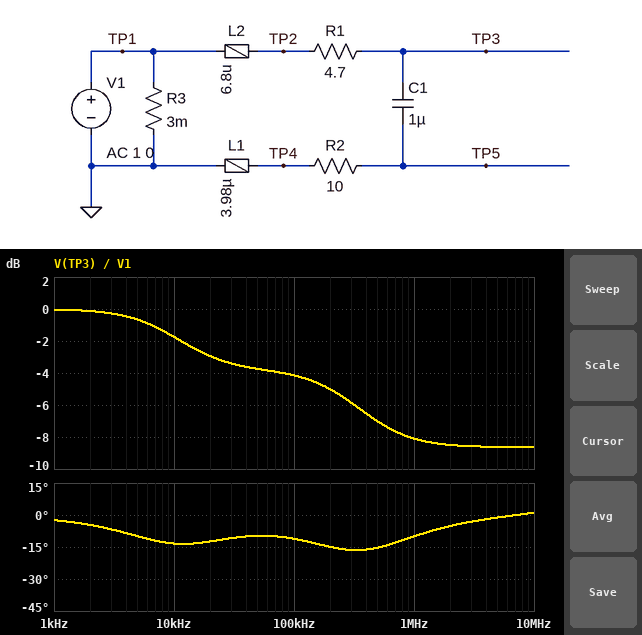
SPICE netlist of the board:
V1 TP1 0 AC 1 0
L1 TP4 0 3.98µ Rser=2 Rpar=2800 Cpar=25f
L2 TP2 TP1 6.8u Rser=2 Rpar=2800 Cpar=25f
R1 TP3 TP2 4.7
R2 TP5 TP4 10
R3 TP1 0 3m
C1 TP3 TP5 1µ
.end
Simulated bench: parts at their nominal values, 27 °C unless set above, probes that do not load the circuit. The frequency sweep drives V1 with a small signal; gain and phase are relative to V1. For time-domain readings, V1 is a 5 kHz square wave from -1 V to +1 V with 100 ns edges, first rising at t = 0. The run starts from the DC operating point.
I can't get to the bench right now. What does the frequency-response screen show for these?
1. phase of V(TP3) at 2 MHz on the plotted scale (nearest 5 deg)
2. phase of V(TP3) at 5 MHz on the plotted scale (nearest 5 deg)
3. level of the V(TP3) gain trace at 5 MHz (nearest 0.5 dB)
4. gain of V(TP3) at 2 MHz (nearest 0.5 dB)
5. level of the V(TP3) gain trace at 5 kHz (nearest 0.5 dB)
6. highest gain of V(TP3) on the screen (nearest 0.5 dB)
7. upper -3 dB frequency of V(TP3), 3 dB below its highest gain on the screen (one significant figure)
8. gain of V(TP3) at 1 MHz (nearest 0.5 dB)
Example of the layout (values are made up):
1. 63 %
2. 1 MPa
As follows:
1. -5 deg
2. 0 deg
3. -8.5 dB
4. -8.5 dB
5. -0.5 dB
6. 0 dB
7. 20 kHz
8. -8.0 dB
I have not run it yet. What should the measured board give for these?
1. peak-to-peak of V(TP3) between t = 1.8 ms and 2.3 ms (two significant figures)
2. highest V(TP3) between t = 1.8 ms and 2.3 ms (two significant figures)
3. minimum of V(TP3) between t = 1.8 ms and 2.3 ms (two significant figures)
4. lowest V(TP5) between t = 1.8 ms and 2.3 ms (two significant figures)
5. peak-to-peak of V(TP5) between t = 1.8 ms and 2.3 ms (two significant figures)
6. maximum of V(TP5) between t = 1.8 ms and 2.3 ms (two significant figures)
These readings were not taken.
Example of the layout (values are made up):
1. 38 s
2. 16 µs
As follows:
1. 2.0 V
2. 1.0 V
3. -1.0 V
4. -1.2 V
5. 2.4 V
6. 1.2 V
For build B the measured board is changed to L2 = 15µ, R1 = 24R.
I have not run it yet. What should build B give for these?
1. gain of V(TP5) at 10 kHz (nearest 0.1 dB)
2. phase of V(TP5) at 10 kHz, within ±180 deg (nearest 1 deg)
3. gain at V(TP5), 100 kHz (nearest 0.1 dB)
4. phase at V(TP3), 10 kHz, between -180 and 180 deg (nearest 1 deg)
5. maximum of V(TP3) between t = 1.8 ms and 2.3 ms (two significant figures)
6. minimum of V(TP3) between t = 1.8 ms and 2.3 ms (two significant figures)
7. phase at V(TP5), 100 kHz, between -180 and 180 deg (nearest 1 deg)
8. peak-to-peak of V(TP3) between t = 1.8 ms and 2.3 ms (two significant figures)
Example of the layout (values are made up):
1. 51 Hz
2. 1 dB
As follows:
1. -10.6 dB
2. 22 deg
3. -10.1 dB
4. -31 deg
5. 910 mV
6. -910 mV
7. -3 deg
8. 1.8 V
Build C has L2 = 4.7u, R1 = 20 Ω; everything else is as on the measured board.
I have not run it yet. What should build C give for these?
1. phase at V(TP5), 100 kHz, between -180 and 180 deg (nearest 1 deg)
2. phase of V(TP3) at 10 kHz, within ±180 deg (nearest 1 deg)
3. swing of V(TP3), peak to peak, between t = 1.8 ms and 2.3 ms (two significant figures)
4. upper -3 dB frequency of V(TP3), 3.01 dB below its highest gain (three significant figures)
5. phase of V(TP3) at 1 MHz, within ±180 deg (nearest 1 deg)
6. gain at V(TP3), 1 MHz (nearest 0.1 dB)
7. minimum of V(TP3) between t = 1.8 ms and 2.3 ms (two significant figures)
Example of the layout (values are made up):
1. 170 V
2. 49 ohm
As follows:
1. 5 deg
2. -28 deg
3. 1.9 V
4. 5.41 kHz
5. 6 deg
6. -7.3 dB
7. -940 mV
